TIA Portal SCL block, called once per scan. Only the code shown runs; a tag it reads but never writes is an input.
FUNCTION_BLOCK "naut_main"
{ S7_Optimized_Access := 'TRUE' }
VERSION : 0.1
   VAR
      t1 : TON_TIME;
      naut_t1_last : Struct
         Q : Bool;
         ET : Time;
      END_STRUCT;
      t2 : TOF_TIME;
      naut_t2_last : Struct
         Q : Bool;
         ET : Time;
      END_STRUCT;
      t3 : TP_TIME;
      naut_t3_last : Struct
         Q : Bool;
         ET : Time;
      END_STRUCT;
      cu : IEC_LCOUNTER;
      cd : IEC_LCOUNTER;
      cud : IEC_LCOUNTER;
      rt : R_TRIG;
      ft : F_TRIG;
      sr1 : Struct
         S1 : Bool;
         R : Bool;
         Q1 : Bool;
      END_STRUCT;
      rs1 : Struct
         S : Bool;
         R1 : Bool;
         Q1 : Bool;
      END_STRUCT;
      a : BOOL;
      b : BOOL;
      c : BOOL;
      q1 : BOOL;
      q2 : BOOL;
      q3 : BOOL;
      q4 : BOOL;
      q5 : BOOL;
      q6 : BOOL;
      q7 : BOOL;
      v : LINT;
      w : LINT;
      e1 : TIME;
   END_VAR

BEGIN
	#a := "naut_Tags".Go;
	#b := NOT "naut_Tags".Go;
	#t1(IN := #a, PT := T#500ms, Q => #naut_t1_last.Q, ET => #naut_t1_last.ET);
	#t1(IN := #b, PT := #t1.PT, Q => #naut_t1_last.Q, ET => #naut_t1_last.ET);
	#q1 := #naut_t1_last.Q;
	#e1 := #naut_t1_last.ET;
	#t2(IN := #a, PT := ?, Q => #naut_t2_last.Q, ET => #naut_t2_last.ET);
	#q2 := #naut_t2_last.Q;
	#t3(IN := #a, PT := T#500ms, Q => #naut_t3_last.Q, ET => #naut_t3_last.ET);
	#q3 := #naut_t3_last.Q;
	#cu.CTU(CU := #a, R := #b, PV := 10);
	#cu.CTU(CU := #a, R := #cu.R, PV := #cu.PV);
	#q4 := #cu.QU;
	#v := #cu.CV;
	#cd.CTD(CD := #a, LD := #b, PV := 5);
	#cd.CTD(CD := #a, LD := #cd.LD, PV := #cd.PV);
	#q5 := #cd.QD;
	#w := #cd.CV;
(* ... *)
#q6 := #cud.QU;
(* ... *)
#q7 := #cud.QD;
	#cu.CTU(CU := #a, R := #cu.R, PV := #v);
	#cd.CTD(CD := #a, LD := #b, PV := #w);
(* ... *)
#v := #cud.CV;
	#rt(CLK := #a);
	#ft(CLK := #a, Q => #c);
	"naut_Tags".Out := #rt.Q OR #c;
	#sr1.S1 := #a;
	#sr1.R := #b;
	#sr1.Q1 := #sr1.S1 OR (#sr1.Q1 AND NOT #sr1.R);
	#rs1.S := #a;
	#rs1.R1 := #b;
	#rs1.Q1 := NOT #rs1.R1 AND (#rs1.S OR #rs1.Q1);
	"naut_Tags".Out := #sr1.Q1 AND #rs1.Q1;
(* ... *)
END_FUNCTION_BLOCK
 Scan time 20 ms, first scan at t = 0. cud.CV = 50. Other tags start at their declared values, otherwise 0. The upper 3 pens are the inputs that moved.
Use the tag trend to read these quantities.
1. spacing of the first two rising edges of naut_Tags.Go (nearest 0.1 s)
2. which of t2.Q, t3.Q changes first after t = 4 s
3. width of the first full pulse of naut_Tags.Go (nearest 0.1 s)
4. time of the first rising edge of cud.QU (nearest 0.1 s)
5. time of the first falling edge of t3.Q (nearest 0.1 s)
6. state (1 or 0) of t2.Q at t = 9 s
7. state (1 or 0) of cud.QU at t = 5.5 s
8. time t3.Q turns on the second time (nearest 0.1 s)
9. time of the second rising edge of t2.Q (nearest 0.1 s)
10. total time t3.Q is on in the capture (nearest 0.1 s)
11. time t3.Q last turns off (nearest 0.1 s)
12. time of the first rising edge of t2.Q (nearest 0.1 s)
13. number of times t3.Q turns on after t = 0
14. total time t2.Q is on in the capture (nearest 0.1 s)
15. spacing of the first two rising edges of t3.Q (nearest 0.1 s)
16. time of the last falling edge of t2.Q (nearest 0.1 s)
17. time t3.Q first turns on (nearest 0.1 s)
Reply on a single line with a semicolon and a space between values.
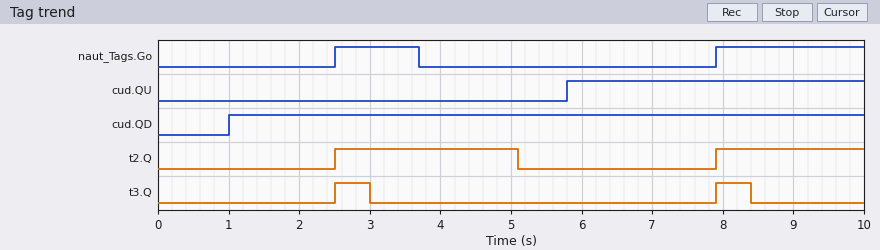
5.4 s; t2.Q; 1.2 s; 5.8 s; 3.0 s; 1; 0; 7.9 s; 7.9 s; 1.0 s; 8.4 s; 2.5 s; 2; 4.7 s; 5.4 s; 5.1 s; 2.5 s
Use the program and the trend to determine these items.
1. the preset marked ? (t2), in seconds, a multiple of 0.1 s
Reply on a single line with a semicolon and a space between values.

1.4 s
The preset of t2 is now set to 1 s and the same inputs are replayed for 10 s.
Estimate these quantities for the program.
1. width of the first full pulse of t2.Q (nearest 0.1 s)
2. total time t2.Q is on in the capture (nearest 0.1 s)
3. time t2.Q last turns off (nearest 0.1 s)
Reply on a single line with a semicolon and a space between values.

2.2 s; 4.3 s; 4.7 s
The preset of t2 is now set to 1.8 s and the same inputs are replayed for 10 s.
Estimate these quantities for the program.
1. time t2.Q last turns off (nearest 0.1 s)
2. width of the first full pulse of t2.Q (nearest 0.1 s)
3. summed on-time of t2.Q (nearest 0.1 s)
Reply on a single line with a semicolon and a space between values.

5.5 s; 3.0 s; 5.1 s
